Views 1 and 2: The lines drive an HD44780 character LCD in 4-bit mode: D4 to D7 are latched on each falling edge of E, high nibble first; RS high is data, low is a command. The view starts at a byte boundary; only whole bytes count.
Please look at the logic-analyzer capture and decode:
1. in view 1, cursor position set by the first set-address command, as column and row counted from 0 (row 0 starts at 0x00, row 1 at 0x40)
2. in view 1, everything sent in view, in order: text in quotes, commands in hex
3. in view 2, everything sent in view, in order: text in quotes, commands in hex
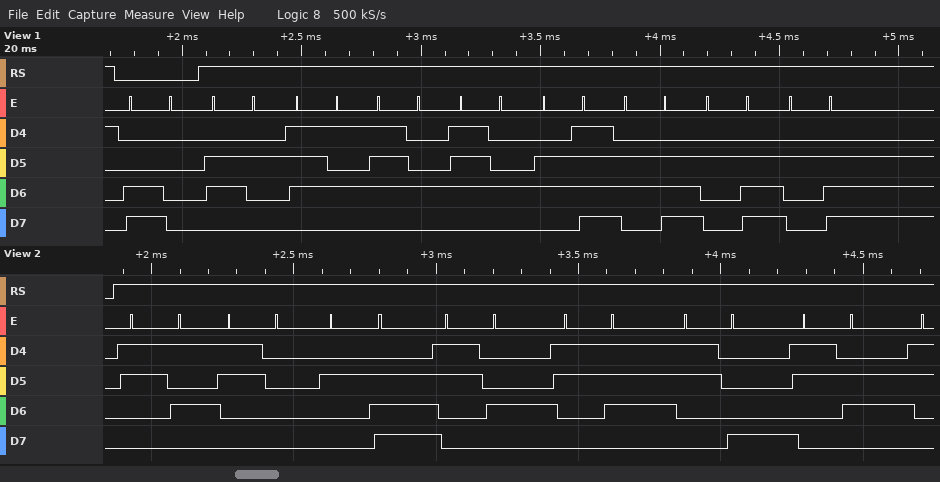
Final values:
column 0, row 1
0xC0 "button.."
"50.4786"
